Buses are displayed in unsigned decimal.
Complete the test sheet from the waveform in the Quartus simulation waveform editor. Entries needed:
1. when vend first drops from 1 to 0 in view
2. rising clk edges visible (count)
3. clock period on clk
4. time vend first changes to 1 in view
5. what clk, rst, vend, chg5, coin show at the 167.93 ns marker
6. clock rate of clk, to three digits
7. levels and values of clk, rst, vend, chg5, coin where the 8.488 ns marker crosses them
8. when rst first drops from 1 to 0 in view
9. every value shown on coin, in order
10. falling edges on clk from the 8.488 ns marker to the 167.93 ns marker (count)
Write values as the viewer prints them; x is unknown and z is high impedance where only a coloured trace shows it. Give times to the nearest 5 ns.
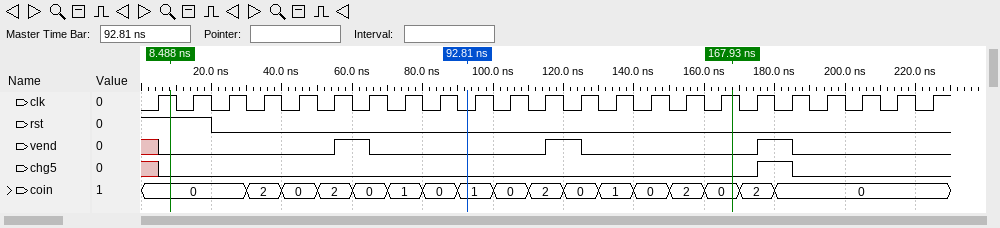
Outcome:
65 ns
23
10 ns
55 ns
clk=1, rst=0, vend=0, chg5=0, coin=0
100 MHz
clk=1, rst=1, vend=0, chg5=0, coin=0
20 ns
0, 2, 0, 2, 0, 1, 0, 1, 0, 2, 0, 1, 0, 2, 0, 2, 0
16
